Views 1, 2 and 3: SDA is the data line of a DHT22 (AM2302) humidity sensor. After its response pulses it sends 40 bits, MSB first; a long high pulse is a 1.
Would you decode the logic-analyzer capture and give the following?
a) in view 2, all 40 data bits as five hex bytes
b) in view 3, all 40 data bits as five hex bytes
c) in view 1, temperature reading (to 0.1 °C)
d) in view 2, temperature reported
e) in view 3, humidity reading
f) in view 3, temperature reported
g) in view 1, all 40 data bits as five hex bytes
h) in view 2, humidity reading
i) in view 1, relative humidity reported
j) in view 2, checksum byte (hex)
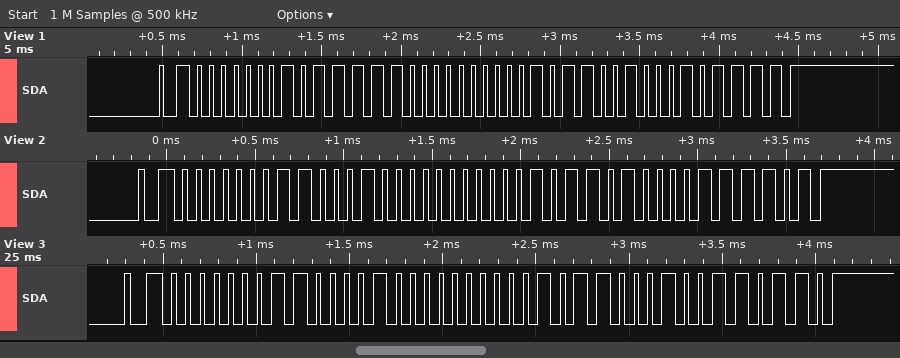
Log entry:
01 88 00 B4 3D
01 84 00 B1 36
17.8 °C
18.0 °C
38.8 %
17.7 °C
01 7C 00 B2 2F
39.2 %
38.0 %
0x3D
